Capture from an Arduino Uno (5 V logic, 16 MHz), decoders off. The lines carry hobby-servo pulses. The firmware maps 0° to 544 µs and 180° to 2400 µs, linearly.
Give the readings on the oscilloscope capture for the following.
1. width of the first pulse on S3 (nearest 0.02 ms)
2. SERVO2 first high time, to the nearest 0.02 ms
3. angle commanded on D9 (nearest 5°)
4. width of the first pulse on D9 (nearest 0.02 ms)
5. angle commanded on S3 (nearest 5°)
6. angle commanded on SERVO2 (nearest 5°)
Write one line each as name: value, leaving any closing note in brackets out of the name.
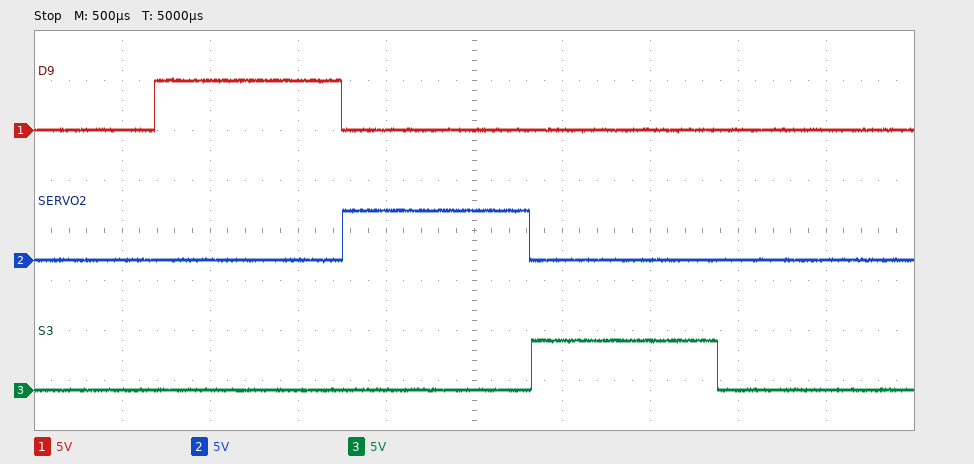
width of the first pulse on S3: 1.06 ms
SERVO2 first high time, to the nearest 0.02 ms: 1.06 ms
angle commanded on D9: 50°
width of the first pulse on D9: 1.06 ms
angle commanded on S3: 50°
angle commanded on SERVO2: 50°
